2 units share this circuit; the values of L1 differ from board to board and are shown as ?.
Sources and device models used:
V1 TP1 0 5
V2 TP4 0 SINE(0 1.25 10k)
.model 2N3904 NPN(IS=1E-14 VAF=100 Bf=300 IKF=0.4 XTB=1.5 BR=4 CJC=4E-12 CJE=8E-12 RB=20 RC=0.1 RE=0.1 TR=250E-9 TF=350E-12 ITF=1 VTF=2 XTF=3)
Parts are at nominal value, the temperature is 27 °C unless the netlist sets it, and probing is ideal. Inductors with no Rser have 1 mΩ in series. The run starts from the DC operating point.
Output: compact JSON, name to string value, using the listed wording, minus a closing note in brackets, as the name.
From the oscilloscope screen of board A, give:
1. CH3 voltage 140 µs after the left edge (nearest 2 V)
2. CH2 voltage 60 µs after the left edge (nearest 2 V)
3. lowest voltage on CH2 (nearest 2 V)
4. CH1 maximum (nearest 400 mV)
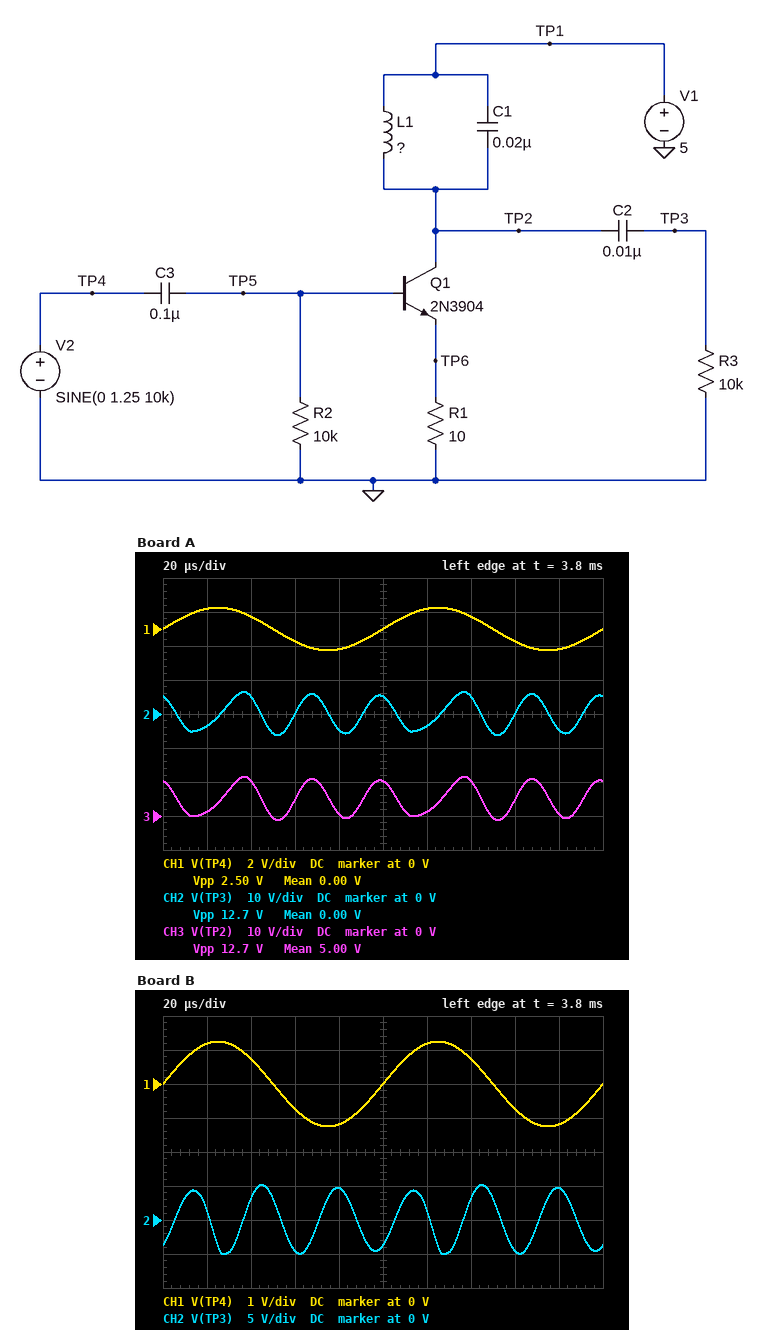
{"CH3 voltage 140 µs after the left edge": "10 V", "CH2 voltage 60 µs after the left edge": "0 V", "lowest voltage on CH2": "-6 V", "CH1 maximum": "1.2 V"}
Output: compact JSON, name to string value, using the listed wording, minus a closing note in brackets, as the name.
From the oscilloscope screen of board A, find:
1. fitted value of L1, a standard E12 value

{"fitted value of L1, a standard E12 value": "1.2 mH"}
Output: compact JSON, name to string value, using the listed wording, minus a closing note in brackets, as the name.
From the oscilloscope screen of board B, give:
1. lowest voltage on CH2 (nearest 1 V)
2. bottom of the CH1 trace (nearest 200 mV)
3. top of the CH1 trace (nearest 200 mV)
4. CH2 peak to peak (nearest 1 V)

{"lowest voltage on CH2": "-5 V", "bottom of the CH1 trace": "-1.2 V", "top of the CH1 trace": "1.2 V", "CH2 peak to peak": "10 V"}
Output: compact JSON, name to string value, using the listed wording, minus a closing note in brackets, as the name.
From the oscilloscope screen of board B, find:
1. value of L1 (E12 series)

{"value of L1": "1.5 mH"}
